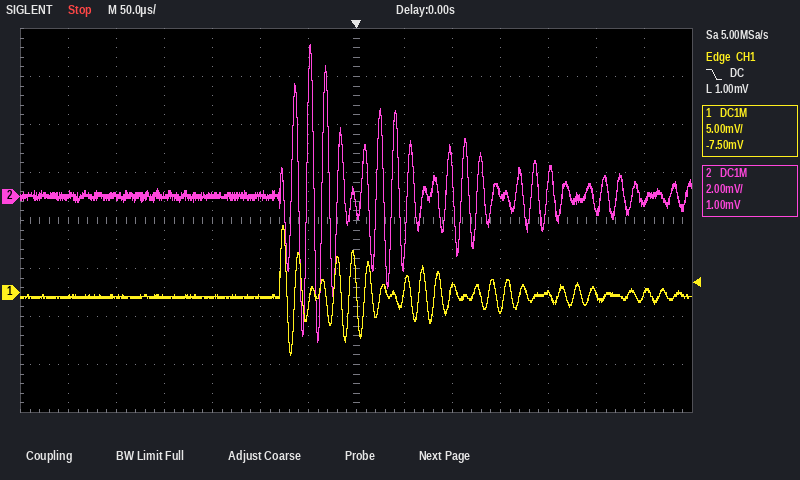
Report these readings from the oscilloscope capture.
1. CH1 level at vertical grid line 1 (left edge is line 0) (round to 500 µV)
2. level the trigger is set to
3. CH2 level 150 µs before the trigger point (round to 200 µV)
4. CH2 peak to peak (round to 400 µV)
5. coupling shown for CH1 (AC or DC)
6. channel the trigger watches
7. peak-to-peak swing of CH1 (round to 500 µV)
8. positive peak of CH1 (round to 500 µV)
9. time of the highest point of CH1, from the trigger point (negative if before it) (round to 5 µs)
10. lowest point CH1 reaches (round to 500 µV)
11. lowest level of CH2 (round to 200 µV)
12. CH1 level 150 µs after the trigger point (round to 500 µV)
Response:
-500 µV
1.00 mV
0.0 mV
12.4 mV
DC
CH1
13.5 mV
7.0 mV
-75 µs
-6.5 mV
-6.0 mV
-2.0 mV
